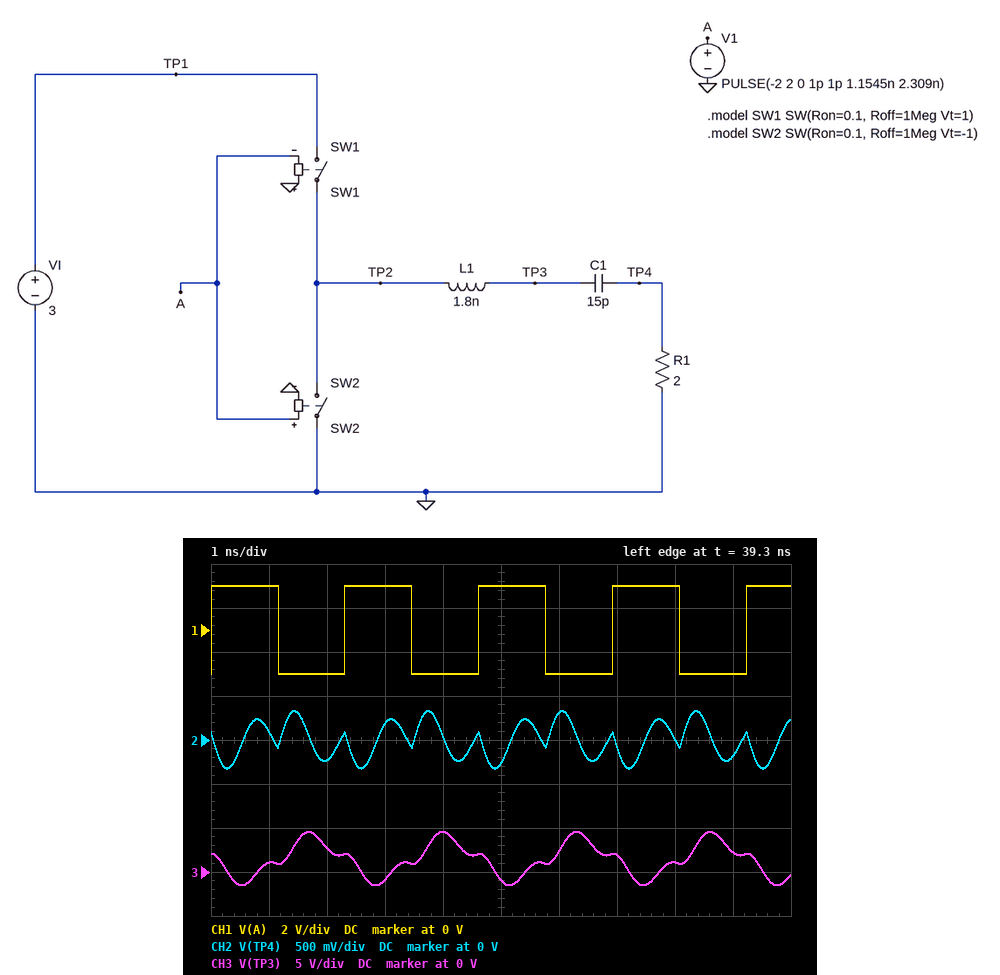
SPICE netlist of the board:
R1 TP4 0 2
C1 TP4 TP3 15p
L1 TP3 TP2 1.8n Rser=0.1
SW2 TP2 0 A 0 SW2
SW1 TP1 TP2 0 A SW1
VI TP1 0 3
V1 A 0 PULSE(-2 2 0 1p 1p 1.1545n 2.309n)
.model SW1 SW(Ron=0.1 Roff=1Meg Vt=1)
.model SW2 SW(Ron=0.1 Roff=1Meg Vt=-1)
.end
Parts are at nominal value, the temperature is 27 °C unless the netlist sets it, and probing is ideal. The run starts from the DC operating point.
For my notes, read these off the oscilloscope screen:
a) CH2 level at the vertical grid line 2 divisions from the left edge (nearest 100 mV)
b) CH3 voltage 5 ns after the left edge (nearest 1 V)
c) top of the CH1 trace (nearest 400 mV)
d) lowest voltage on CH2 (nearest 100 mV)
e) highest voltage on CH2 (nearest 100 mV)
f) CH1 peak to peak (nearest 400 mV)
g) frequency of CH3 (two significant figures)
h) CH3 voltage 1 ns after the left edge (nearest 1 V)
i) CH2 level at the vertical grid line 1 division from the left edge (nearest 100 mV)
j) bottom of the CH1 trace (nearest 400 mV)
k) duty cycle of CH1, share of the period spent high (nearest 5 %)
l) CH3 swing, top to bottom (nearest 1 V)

-200 mV
-1 V
2.0 V
-300 mV
300 mV
4.0 V
430 MHz
1 V
100 mV
-2.0 V
50 %
6 V
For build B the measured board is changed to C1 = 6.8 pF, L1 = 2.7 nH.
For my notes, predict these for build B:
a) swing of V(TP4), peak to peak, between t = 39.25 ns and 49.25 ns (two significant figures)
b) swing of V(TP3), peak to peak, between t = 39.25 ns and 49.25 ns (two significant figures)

670 mV
9.1 V
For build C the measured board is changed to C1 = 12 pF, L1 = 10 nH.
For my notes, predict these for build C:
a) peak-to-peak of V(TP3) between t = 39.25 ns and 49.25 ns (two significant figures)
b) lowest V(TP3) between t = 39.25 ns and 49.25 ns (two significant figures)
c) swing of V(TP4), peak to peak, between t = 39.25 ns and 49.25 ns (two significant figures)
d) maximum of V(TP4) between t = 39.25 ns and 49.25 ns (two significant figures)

29 V
-13 V
1.9 V
950 mV
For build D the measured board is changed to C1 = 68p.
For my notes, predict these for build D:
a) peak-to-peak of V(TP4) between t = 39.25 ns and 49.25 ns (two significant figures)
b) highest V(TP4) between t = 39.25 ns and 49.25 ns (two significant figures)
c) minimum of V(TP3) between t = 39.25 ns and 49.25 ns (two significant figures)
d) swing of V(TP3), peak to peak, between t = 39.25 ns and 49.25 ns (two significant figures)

3.5 V
1.7 V
-3.3 V
9.5 V
